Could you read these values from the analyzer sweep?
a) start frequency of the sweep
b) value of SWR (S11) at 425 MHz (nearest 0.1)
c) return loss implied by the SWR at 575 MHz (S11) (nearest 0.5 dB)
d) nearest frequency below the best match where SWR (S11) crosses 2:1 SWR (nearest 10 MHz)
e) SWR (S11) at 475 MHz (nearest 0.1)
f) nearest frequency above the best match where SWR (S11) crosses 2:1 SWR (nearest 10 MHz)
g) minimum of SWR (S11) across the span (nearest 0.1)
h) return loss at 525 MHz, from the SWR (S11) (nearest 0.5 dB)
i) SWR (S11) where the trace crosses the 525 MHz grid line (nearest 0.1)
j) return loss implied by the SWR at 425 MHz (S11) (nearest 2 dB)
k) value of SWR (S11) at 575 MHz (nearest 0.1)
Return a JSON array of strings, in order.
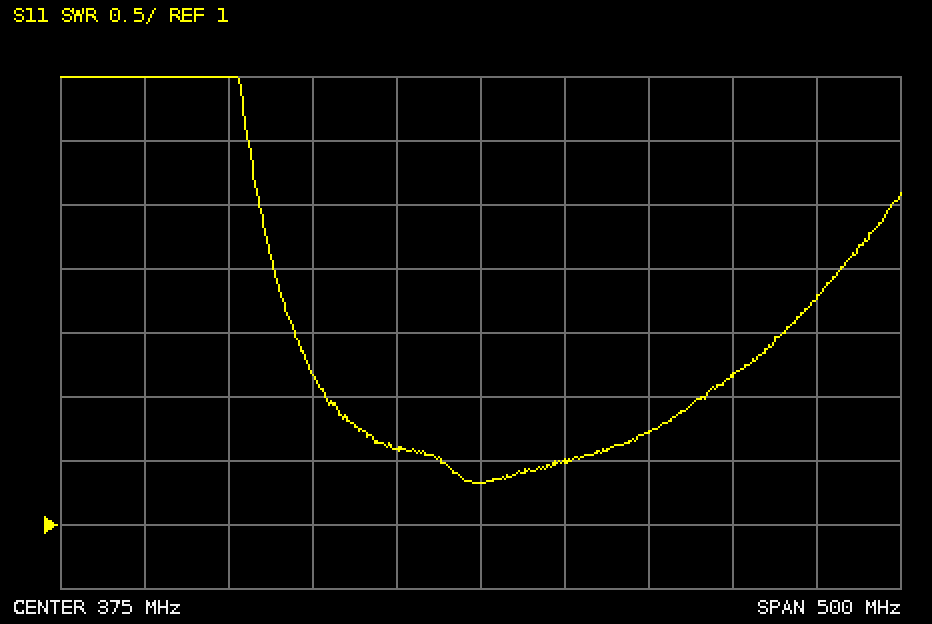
["125 MHz", "1.5", "6.5 dB", "280 MHz", "1.7", "510 MHz", "1.3", "8.5 dB", "2.2", "14 dB", "2.8"]
